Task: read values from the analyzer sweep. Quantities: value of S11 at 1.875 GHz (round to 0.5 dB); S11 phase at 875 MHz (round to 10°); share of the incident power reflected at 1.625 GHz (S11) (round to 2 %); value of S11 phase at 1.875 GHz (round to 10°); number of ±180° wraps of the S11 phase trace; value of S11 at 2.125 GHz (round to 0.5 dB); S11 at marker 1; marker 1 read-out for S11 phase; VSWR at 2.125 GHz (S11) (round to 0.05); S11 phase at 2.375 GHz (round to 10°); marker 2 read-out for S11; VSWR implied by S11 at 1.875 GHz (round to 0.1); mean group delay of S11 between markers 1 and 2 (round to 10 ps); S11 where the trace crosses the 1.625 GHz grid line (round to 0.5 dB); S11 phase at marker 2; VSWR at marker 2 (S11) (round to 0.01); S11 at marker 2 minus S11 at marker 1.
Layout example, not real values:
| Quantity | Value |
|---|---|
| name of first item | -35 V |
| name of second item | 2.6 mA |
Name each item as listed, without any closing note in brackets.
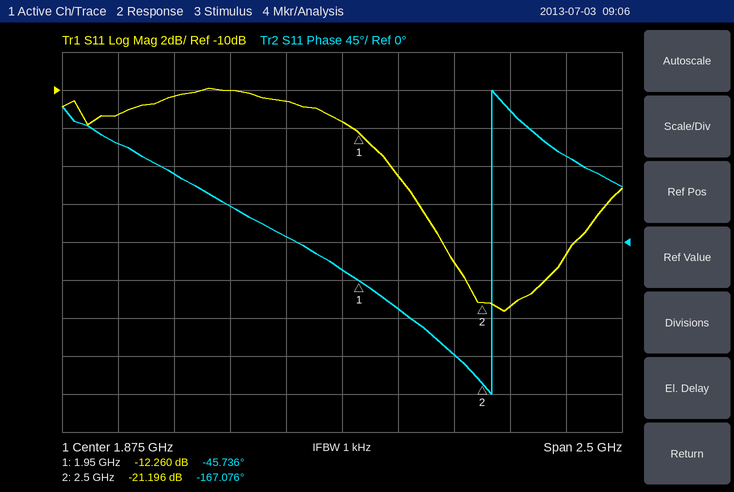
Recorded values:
| Quantity | Value |
|---|---|
| value of S11 at 1.875 GHz | -11.5 dB |
| S11 phase at 875 MHz | 120° |
| share of the incident power reflected at 1.625 GHz (S11) | 8 % |
| value of S11 phase at 1.875 GHz | -30° |
| number of ±180° wraps of the S11 phase trace | 1 |
| value of S11 at 2.125 GHz | -14.5 dB |
| S11 at marker 1 | -12.260 dB |
| marker 1 read-out for S11 phase | -45.736° |
| VSWR at 2.125 GHz (S11) | 1.45 |
| S11 phase at 2.375 GHz | -130° |
| marker 2 read-out for S11 | -21.196 dB |
| VSWR implied by S11 at 1.875 GHz | 1.7 |
| mean group delay of S11 between markers 1 and 2 | 610 ps |
| S11 where the trace crosses the 1.625 GHz grid line | -10.5 dB |
| S11 phase at marker 2 | -167.076° |
| VSWR at marker 2 (S11) | 1.19 |
| S11 at marker 2 minus S11 at marker 1 | -8.936 dB |
